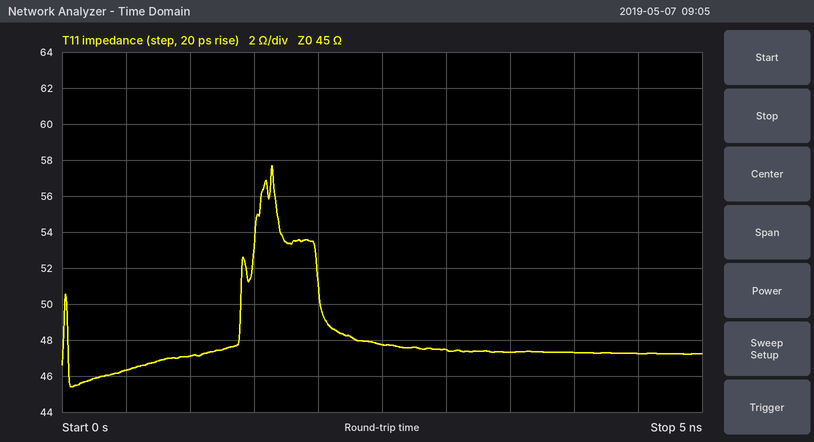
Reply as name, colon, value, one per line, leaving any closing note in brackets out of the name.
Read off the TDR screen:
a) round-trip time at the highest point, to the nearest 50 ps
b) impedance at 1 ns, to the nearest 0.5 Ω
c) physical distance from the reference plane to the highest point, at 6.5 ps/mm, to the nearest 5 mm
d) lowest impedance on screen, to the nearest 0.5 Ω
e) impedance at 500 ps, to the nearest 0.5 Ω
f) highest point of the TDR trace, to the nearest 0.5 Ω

round-trip time at the highest point, to the nearest 50 ps: 1.65 ns
impedance at 1 ns, to the nearest 0.5 Ω: 47.0 Ω
physical distance from the reference plane to the highest point, at 6.5 ps/mm, to the nearest 5 mm: 125 mm
lowest impedance on screen, to the nearest 0.5 Ω: 45.5 Ω
impedance at 500 ps, to the nearest 0.5 Ω: 46.5 Ω
highest point of the TDR trace, to the nearest 0.5 Ω: 57.5 Ω
